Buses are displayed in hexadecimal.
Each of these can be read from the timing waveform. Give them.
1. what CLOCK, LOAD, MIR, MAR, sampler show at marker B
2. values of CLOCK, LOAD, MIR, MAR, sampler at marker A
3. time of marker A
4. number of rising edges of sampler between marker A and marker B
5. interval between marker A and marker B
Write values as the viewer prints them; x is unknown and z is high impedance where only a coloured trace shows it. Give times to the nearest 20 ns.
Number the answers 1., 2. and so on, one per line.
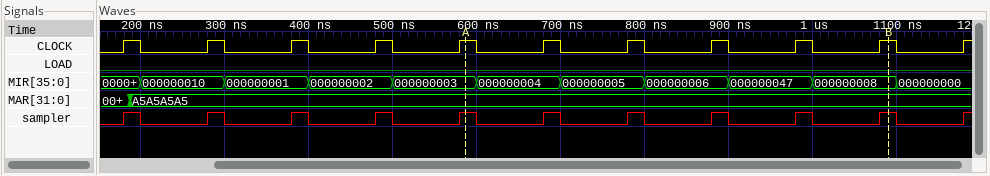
1. CLOCK=1, LOAD=0, MIR=000000008, MAR=A5A5A5A5, sampler=1
2. CLOCK=1, LOAD=0, MIR=000000003, MAR=A5A5A5A5, sampler=1
3. 580 ns
4. 5
5. 500 ns
